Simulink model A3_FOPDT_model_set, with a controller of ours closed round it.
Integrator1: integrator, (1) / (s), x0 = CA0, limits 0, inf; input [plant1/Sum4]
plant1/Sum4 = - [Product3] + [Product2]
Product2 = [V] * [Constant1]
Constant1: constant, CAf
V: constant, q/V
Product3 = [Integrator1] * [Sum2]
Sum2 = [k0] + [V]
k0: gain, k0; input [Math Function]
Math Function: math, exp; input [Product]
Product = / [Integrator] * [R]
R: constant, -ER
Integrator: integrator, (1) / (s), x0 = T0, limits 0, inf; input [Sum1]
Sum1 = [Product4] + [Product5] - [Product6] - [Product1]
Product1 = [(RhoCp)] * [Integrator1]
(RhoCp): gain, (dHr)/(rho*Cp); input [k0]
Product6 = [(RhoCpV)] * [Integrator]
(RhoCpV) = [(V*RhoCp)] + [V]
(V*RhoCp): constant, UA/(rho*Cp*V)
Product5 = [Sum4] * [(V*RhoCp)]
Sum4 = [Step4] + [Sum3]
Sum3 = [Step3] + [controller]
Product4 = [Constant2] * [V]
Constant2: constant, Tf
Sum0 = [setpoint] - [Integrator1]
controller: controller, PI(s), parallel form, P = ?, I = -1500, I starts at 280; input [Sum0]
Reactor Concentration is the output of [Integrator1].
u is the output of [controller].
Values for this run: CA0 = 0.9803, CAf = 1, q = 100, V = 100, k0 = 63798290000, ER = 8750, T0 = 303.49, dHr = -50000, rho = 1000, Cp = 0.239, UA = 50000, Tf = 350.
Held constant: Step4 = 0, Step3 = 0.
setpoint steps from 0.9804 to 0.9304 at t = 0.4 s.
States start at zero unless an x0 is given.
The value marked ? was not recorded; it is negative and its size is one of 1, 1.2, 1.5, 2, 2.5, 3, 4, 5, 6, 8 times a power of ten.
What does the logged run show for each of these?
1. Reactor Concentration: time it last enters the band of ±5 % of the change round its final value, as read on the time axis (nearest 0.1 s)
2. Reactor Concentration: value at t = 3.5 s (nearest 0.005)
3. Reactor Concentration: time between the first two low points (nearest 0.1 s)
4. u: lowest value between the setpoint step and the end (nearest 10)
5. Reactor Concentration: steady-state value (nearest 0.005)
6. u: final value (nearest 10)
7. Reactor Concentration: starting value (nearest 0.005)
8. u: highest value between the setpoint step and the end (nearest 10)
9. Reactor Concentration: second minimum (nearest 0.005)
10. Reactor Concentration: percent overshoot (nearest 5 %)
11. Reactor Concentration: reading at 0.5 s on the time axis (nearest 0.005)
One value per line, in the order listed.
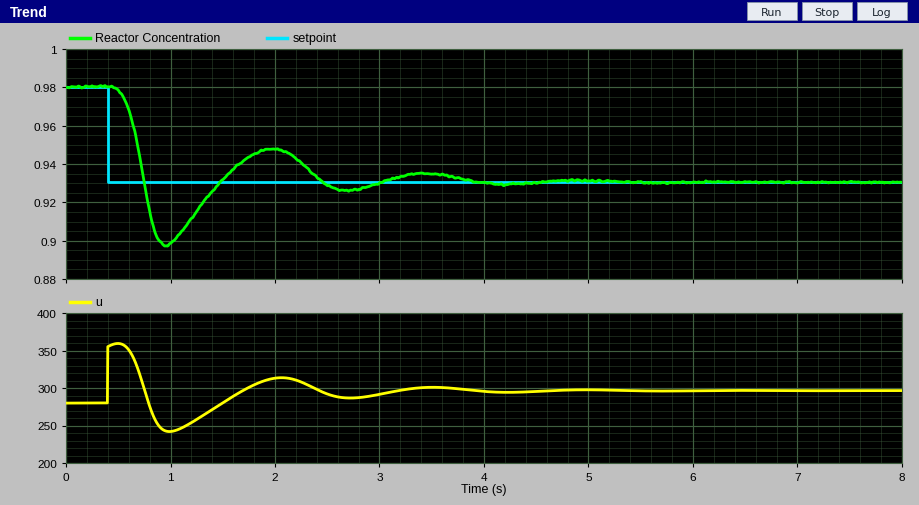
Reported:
3.7 s
0.935
1.7 s
240
0.930
300
0.980
360
0.925
65 %
0.980
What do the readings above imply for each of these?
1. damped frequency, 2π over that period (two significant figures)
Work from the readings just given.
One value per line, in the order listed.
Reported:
3.7 rad/s
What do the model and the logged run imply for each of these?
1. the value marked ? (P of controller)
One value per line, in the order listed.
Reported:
-1500
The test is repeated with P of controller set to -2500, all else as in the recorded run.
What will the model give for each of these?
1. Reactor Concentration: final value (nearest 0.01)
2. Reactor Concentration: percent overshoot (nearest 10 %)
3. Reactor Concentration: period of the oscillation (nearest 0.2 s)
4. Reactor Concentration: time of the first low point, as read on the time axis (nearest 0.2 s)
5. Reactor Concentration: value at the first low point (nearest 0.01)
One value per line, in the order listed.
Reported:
0.93
80 %
1.4 s
0.8 s
0.89
